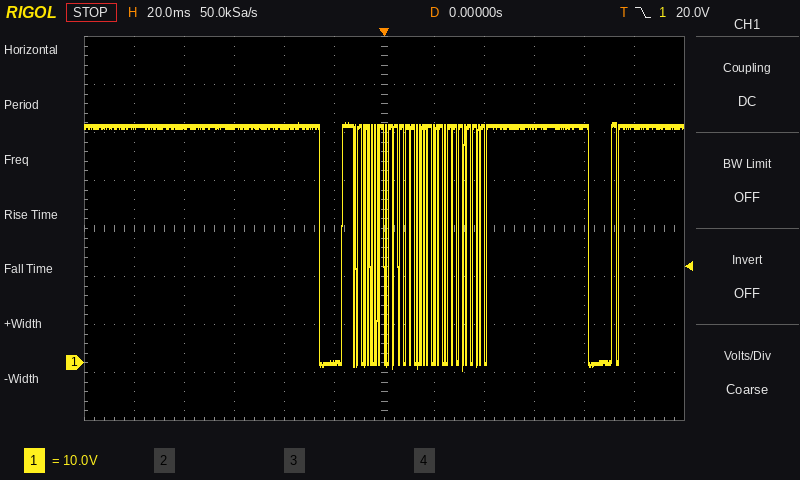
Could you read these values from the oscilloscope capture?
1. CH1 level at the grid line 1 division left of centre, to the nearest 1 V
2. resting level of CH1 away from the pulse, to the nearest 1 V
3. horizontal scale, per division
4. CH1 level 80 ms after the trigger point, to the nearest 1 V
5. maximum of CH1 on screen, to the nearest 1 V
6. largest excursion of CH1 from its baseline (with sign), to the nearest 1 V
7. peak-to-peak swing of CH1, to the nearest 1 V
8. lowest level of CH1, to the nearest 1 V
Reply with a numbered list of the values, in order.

1. 0 V
2. 49 V
3. 20 ms
4. 49 V
5. 50 V
6. -51 V
7. 52 V
8. -2 V
